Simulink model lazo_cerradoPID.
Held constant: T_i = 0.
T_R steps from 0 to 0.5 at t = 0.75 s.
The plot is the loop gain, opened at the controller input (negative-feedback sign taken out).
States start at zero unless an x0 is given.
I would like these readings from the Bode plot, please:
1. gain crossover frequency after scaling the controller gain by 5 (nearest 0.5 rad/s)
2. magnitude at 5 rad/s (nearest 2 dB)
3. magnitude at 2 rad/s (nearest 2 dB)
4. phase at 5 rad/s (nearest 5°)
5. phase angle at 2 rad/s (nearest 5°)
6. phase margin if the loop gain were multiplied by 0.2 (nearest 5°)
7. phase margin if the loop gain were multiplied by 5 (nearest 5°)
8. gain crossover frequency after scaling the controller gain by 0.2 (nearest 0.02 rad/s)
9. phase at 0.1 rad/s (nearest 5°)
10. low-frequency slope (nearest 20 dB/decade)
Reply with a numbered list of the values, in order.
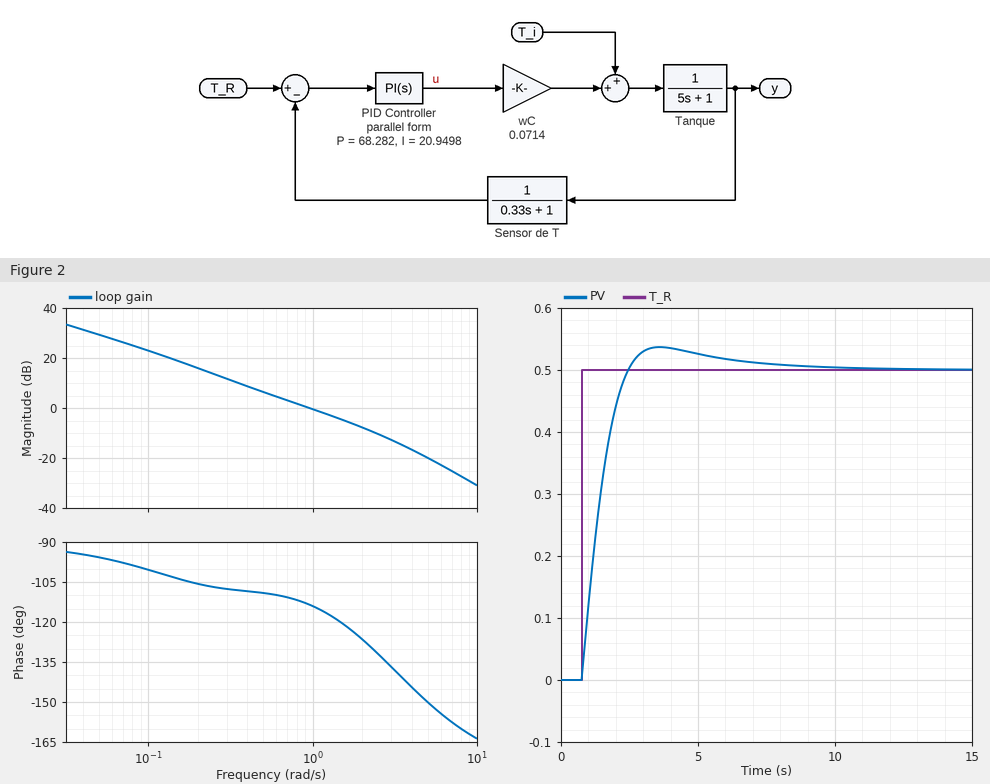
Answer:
1. 3.5 rad/s
2. -20 dB
3. -8 dB
4. -150°
5. -125°
6. 75°
7. 40°
8. 0.24 rad/s
9. -100°
10. -20 dB/decade
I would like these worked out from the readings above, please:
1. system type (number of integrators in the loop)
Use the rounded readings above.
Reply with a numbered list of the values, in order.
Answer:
1. 1
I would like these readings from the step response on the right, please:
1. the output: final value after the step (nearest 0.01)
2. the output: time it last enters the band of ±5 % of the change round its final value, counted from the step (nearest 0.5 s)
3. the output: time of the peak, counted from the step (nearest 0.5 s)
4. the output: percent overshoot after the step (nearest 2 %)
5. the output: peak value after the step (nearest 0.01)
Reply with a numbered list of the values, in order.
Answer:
1. 0.50
2. 4.5 s
3. 3.0 s
4. 8 %
5. 0.54
